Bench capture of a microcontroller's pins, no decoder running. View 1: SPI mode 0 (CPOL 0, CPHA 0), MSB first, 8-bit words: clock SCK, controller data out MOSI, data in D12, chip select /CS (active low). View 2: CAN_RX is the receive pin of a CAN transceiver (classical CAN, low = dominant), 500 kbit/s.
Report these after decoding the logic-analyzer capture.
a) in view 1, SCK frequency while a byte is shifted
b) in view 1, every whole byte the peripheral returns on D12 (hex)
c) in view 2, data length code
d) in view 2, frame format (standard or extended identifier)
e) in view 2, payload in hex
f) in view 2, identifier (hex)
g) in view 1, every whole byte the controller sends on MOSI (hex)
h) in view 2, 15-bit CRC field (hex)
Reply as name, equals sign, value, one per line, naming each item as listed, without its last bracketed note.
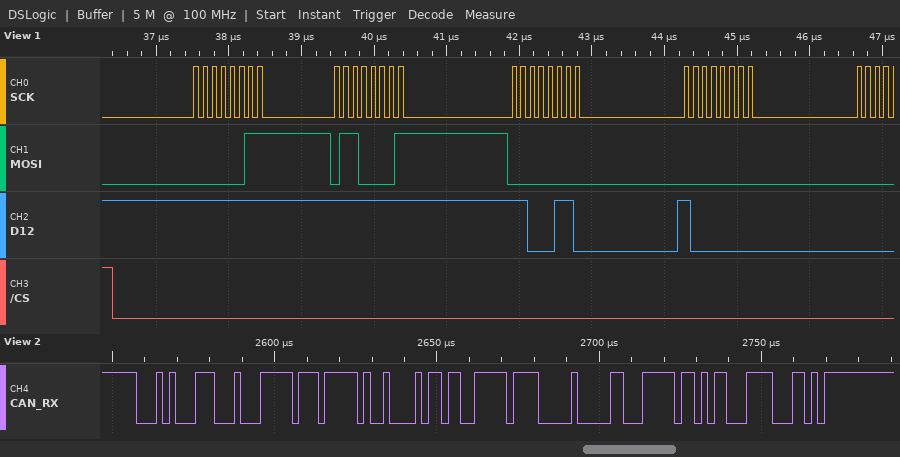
in view 1, SCK frequency while a byte is shifted = 8 MHz
in view 1, every whole byte the peripheral returns on D12 = FF FF C6 80
in view 2, data length code = 8
in view 2, frame format = standard
in view 2, payload in hex = FF 7E 42 D9 FF 00 23 FA
in view 2, identifier = 0x147
in view 1, every whole byte the controller sends on MOSI = 03 61 00 00
in view 2, 15-bit CRC field = 0x63C6
